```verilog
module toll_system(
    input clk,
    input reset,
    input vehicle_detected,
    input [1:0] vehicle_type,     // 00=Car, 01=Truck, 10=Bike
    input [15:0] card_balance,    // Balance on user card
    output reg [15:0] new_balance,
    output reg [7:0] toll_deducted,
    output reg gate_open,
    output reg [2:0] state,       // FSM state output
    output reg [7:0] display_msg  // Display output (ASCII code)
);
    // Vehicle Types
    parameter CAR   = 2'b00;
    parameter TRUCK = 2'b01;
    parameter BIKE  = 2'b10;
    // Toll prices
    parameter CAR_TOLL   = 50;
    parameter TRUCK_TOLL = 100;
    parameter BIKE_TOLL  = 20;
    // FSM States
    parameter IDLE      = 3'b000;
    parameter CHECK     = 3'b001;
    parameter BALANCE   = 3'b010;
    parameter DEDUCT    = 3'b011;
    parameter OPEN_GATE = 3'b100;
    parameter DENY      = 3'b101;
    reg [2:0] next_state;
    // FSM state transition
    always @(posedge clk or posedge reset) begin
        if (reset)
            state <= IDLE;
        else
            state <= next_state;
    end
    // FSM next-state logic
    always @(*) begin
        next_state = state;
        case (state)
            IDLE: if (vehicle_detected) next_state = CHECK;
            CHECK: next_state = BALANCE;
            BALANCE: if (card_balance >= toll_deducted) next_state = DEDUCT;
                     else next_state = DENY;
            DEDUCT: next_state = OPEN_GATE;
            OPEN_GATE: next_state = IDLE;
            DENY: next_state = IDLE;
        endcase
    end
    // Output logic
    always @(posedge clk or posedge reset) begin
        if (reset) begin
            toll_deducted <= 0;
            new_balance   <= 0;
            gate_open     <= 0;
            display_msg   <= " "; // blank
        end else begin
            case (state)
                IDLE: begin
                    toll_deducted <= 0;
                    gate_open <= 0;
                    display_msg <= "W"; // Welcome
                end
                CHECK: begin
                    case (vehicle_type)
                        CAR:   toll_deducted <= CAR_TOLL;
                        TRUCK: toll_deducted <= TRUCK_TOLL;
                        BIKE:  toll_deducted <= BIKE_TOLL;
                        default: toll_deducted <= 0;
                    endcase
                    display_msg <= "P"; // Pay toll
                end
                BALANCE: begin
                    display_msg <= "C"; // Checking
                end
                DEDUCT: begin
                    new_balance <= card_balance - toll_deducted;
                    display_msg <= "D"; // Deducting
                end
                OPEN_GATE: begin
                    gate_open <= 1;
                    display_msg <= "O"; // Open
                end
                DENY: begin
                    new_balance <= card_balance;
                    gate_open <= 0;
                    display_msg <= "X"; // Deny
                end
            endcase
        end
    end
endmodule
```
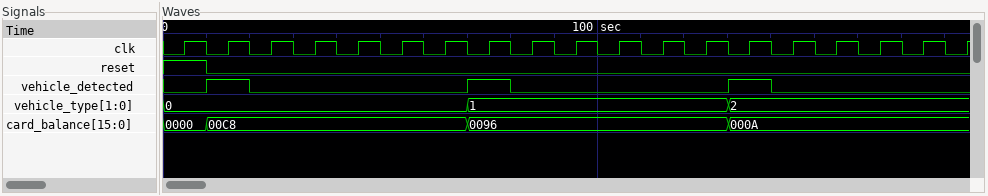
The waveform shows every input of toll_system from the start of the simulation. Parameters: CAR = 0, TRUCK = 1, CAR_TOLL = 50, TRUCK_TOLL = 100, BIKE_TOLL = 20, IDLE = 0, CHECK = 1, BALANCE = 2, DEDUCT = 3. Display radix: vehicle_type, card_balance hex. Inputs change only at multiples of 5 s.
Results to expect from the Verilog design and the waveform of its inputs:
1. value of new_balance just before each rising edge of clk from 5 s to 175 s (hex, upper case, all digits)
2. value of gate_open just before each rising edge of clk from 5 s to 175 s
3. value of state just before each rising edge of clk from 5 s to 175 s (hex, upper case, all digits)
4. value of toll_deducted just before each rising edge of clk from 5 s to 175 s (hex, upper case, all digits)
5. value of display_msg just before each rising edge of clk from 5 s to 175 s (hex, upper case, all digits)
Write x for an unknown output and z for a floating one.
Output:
0000, 0000, 0000, 0000, 0000, 0096, 0096, 0096, 0096, 0096, 0096, 0032, 0032, 0032, 0032, 0032, 0032, 000A
0 0 0 0 0 0 1 0 0 0 0 0 1 0 0 0 0 0
0, 0, 1, 2, 3, 4, 0, 0, 1, 2, 3, 4, 0, 0, 1, 2, 5, 0
00, 00, 00, 32, 32, 32, 32, 00, 00, 64, 64, 64, 64, 00, 00, 14, 14, 14
20, 20, 57, 50, 43, 44, 4F, 57, 57, 50, 43, 44, 4F, 57, 57, 50, 43, 58
